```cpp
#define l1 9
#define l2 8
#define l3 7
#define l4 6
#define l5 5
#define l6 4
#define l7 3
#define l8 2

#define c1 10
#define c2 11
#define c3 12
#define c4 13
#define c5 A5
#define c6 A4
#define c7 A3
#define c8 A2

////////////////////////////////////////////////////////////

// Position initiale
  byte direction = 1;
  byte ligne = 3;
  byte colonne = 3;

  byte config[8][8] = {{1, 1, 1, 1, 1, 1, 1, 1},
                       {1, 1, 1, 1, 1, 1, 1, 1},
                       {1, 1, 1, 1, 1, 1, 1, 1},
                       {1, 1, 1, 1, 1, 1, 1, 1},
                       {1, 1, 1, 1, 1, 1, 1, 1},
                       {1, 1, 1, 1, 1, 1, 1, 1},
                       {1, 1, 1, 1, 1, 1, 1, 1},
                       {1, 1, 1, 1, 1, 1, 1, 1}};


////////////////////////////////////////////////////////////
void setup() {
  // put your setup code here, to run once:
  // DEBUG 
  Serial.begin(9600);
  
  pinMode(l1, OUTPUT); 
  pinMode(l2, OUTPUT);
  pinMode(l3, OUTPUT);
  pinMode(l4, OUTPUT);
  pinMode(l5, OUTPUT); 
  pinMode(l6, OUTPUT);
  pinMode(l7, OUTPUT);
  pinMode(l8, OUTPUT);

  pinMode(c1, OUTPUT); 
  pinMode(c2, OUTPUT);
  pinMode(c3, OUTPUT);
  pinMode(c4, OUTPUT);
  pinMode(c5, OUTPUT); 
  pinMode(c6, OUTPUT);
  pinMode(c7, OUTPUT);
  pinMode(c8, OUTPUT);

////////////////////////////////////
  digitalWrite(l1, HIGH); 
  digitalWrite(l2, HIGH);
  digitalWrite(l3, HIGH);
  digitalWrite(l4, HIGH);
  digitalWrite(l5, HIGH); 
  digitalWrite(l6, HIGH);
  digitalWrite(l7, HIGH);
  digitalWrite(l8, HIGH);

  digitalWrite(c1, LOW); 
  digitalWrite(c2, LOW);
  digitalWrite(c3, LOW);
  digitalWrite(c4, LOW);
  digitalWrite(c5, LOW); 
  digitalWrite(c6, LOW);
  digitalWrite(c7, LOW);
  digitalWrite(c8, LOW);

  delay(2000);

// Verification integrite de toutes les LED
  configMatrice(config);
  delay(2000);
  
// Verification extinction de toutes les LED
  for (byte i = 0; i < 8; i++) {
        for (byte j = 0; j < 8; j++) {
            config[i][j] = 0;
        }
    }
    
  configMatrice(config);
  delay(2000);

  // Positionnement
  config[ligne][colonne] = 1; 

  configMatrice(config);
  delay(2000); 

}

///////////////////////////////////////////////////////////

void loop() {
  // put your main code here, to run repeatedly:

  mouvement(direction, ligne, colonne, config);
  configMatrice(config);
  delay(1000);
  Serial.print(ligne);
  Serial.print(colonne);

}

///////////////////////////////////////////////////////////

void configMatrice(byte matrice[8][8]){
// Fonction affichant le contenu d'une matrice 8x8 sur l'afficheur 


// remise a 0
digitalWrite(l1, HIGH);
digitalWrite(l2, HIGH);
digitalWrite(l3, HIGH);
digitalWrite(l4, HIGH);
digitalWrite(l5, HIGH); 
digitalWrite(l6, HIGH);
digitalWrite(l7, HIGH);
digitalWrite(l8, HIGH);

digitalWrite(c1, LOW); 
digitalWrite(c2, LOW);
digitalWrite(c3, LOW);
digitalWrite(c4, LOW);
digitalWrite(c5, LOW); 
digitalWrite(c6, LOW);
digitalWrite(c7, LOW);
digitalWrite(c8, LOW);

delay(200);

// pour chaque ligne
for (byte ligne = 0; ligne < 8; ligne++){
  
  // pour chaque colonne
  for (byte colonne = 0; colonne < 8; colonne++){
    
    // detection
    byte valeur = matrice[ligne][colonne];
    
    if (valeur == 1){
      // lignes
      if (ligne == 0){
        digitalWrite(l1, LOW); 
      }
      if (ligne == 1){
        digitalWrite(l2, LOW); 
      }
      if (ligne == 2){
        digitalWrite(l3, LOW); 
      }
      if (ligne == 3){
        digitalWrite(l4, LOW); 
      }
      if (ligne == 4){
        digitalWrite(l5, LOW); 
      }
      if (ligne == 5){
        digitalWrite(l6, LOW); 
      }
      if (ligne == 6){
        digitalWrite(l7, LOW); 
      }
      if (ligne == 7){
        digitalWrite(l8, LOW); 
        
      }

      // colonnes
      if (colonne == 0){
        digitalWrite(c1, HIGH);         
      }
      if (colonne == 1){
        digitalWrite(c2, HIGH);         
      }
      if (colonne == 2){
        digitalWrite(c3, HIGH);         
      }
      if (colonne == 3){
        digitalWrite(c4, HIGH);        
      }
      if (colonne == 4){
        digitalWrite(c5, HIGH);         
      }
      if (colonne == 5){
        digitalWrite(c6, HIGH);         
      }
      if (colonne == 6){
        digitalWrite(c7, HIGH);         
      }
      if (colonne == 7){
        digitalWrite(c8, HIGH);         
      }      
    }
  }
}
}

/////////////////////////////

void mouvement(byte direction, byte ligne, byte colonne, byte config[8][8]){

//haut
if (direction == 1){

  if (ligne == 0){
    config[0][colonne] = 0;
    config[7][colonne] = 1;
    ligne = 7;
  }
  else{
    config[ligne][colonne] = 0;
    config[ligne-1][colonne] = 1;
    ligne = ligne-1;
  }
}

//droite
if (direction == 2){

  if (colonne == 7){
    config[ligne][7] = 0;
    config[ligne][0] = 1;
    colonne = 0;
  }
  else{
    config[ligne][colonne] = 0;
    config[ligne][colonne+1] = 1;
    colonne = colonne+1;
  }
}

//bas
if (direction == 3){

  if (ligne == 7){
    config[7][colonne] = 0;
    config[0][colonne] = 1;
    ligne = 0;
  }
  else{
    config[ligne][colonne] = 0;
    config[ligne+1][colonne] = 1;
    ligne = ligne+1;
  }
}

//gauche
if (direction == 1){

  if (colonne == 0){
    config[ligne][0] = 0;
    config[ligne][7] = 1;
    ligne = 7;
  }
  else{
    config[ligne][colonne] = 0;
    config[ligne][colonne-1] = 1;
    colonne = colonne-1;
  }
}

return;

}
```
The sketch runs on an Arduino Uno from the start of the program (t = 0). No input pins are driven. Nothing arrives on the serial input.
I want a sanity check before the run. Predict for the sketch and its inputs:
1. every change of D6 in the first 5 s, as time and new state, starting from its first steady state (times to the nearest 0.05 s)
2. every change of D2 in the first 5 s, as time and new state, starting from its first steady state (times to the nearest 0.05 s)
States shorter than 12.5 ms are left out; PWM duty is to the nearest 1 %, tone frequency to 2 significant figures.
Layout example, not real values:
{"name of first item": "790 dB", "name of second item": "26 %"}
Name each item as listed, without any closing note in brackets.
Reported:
{"every change of D6 in the first 5 s, as time and new state, starting from its first steady state": "0 s high; 2.2 s low; 4.2 s high", "every change of D2 in the first 5 s, as time and new state, starting from its first steady state": "0 s high; 2.2 s low; 4.2 s high"}
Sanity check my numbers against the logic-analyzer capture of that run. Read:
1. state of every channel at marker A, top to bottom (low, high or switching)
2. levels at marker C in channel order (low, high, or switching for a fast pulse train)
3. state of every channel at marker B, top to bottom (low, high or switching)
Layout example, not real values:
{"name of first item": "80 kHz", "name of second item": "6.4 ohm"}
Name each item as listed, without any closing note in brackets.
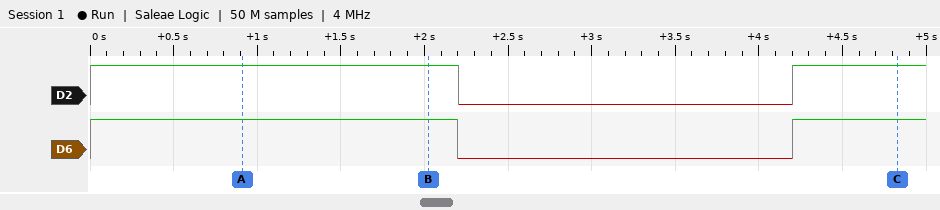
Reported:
{"state of every channel at marker A, top to bottom": "D2 high, D6 high", "levels at marker C in channel order": "D2 high, D6 high", "state of every channel at marker B, top to bottom": "D2 high, D6 high"}
